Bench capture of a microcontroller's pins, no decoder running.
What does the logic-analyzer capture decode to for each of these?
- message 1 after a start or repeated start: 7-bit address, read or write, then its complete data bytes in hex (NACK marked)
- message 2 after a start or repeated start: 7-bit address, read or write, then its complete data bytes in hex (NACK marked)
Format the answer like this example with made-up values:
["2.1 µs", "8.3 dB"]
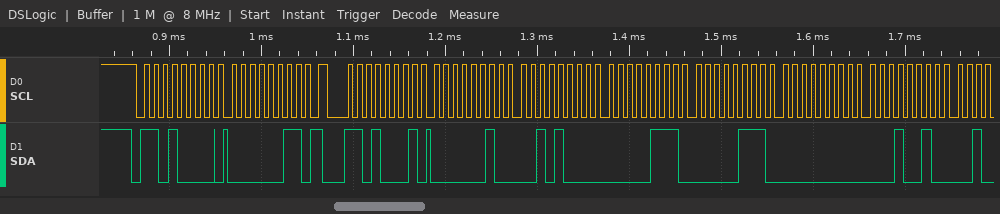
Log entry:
["0x68 write: 03", "0x68 read: 02 28 07 07 00 12"]
